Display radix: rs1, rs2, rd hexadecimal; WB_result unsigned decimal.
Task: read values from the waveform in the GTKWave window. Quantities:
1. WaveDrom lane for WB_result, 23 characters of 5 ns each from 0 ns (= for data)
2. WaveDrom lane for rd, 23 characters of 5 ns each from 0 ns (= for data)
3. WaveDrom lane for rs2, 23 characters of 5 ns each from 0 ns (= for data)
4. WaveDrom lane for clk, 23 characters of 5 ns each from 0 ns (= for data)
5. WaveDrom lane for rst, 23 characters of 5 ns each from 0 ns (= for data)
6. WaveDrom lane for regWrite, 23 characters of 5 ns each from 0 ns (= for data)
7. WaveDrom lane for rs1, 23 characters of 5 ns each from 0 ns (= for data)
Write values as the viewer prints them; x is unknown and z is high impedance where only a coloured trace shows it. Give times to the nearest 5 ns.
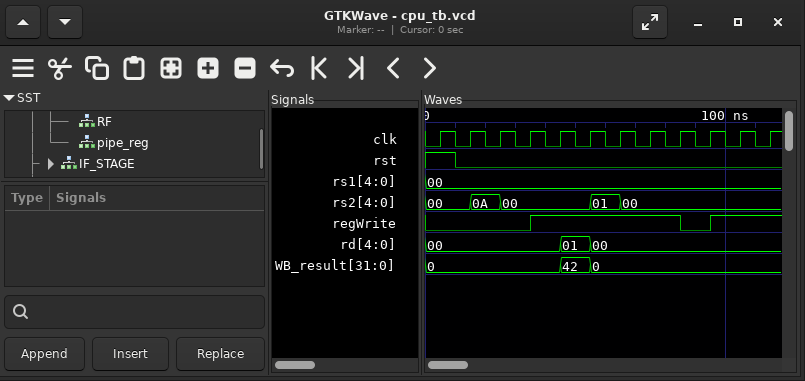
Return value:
{name: 'WB_result', wave: '=........=.=...........', data: '0 42 0'}
{name: 'rd', wave: '=........=.=...........', data: '00 01 00'}
{name: 'rs2', wave: '=..=.=.....=.=.........', data: '00 0A 00 01 00'}
{name: 'clk', wave: '01010101010101010101010'}
{name: 'rst', wave: '1.0....................'}
{name: 'regWrite', wave: '0......1.........0.1...'}
{name: 'rs1', wave: '=......................', data: '00'}
